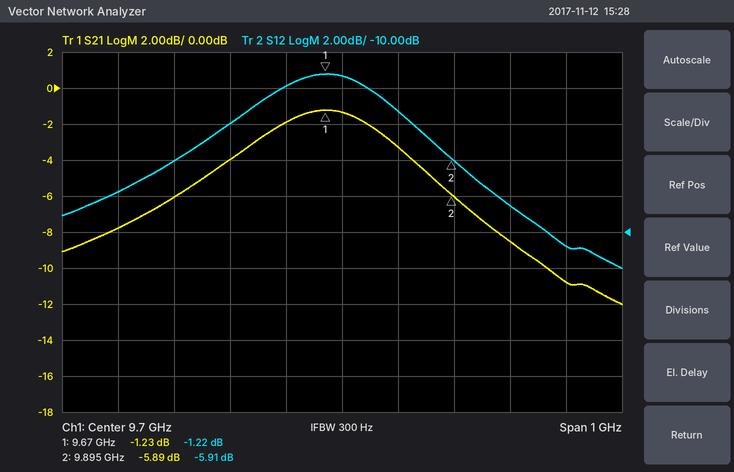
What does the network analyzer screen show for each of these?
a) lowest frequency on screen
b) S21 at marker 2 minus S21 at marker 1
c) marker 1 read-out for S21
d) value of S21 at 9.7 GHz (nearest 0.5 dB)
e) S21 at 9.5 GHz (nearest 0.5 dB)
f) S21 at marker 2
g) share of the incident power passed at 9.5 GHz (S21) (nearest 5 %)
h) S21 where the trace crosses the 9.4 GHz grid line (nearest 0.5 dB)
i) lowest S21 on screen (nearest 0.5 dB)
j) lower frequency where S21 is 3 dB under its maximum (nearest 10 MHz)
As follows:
9.2 GHz
-4.66 dB
-1.23 dB
-1.5 dB
-4.0 dB
-5.89 dB
40 %
-6.0 dB
-12.0 dB
9.49 GHz
